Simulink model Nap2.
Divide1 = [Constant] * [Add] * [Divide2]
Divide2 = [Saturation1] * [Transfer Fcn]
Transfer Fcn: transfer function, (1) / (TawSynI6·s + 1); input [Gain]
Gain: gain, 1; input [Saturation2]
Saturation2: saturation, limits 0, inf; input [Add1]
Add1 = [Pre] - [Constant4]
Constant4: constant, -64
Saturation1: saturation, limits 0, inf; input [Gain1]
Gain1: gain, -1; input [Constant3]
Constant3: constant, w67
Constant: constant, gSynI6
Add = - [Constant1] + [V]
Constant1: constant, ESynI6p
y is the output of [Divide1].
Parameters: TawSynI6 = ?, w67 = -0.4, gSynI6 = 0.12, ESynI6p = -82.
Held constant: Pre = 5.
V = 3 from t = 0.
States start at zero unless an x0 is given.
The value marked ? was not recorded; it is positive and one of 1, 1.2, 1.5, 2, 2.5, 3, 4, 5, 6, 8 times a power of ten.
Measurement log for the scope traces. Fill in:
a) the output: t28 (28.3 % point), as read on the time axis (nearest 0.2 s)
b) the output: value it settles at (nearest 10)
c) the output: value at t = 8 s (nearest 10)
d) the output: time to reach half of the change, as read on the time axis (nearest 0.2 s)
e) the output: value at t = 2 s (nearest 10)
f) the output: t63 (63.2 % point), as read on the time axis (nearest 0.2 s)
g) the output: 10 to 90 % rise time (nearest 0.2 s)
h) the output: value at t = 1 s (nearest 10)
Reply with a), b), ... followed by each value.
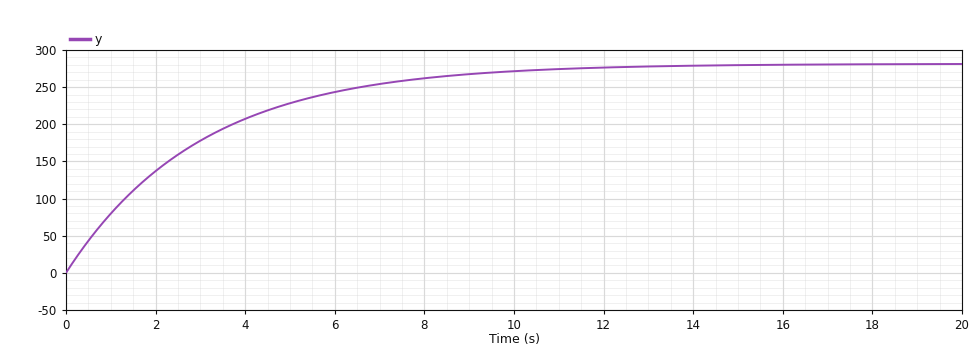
a) 1.0 s
b) 280
c) 260
d) 2.0 s
e) 140
f) 3.0 s
g) 6.6 s
h) 80
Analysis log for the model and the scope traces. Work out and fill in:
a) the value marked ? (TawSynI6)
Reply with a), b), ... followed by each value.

a) 3
